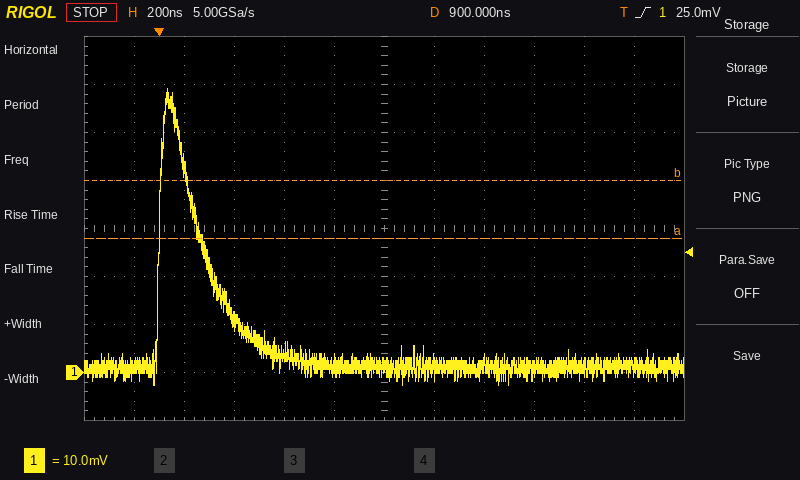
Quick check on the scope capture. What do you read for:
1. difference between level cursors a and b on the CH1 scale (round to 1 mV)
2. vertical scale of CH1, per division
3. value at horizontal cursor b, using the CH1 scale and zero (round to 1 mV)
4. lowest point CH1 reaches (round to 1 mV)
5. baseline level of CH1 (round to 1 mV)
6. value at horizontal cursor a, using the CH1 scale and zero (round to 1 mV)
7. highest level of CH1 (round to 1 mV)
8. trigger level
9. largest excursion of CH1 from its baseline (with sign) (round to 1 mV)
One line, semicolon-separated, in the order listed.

12 mV; 10 mV; 40 mV; -2 mV; 1 mV; 28 mV; 59 mV; 25.0 mV; +58 mV
